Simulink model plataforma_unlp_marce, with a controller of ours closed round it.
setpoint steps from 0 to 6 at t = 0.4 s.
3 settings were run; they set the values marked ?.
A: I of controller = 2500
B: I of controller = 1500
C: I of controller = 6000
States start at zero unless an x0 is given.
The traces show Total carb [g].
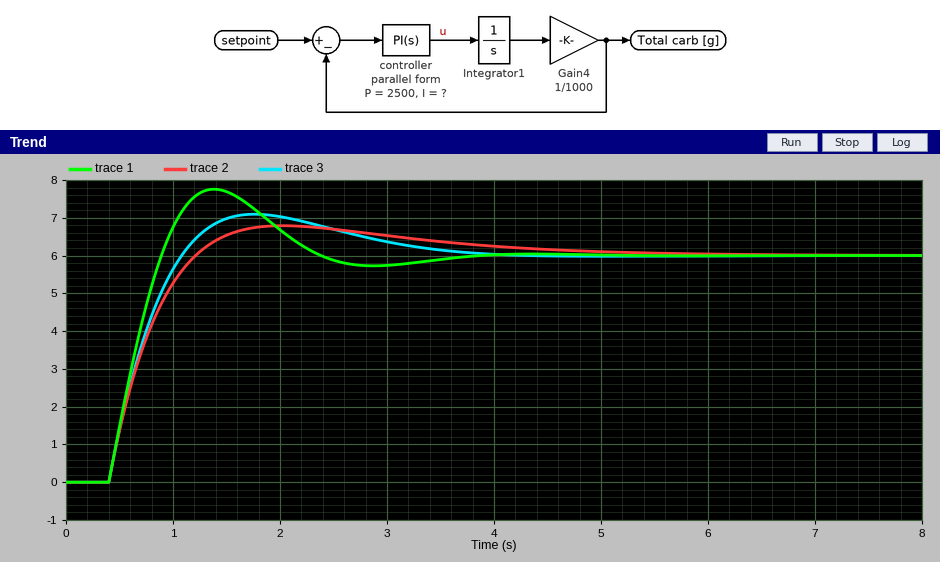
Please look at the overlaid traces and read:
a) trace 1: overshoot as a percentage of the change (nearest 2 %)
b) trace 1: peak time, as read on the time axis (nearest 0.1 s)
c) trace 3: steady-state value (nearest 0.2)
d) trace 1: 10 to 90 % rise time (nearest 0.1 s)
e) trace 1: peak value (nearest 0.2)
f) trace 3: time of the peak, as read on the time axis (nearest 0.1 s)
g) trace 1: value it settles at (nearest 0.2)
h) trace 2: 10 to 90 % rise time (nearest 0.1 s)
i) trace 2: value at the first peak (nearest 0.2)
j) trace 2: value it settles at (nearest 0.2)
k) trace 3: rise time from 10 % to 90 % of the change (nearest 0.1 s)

30 %
1.4 s
6.0
0.4 s
7.8
1.8 s
6.0
0.6 s
6.8
6.0
0.5 s
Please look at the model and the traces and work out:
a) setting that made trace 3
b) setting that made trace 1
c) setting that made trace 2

A
C
B
